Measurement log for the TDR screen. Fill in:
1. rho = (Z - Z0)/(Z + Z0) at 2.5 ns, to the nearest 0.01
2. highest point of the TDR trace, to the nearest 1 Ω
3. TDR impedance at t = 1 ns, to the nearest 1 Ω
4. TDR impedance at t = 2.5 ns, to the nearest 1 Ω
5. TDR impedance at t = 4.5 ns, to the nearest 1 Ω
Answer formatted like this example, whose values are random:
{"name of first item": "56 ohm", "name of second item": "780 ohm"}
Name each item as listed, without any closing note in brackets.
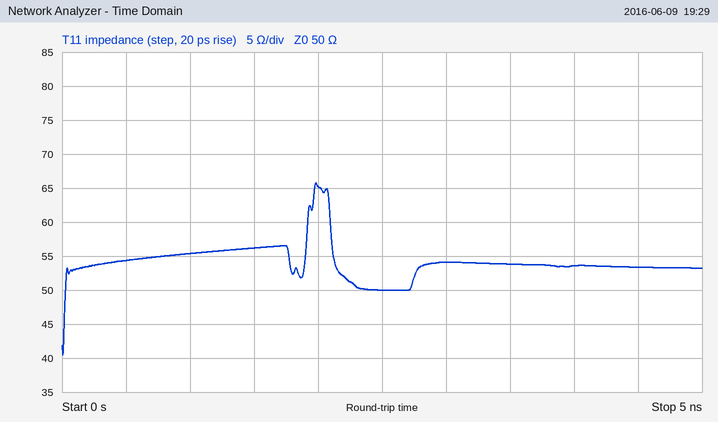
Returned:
{"rho = (Z - Z0)/(Z + Z0) at 2.5 ns, to the nearest 0.01": "0.00", "highest point of the TDR trace, to the nearest 1 Ω": "66 Ω", "TDR impedance at t = 1 ns, to the nearest 1 Ω": "55 Ω", "TDR impedance at t = 2.5 ns, to the nearest 1 Ω": "50 Ω", "TDR impedance at t = 4.5 ns, to the nearest 1 Ω": "53 Ω"}
